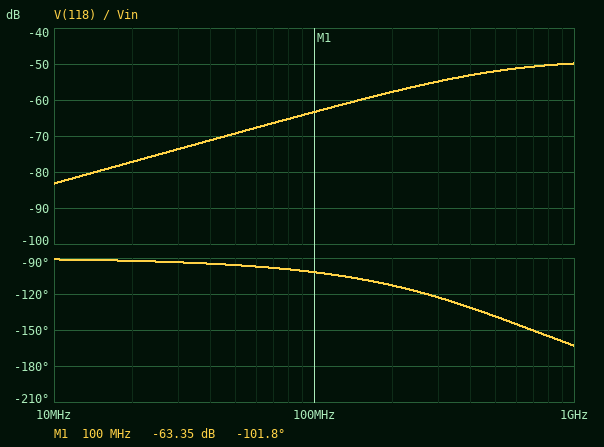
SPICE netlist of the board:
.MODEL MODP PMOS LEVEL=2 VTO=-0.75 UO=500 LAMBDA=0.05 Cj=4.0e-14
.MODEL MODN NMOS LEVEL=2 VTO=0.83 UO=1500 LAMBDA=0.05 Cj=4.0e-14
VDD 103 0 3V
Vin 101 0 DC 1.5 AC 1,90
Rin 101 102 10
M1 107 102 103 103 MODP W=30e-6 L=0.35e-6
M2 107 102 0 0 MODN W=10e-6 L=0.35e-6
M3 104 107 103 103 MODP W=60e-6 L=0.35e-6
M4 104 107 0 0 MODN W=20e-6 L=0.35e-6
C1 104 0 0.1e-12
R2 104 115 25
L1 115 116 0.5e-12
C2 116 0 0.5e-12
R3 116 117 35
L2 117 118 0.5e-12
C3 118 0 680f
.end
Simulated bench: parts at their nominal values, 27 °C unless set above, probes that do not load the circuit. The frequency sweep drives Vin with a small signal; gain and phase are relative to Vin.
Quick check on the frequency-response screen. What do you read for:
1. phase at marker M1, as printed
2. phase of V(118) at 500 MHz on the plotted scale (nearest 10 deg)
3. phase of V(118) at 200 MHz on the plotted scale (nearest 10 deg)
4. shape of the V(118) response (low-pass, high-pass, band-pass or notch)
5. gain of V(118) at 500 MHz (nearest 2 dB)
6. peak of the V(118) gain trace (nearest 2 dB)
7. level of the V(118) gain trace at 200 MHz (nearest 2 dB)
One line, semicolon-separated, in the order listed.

-101.8 deg; -140 deg; -110 deg; high-pass; -52 dB; -50 dB; -58 dB
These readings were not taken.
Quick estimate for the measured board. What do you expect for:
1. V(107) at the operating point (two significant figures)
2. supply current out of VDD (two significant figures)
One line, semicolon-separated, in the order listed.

2.5 V; 380 µA
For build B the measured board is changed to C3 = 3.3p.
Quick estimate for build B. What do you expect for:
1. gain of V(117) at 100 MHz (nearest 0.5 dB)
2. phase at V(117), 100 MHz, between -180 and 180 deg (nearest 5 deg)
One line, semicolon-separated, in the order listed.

-64.5 dB; -125 deg
